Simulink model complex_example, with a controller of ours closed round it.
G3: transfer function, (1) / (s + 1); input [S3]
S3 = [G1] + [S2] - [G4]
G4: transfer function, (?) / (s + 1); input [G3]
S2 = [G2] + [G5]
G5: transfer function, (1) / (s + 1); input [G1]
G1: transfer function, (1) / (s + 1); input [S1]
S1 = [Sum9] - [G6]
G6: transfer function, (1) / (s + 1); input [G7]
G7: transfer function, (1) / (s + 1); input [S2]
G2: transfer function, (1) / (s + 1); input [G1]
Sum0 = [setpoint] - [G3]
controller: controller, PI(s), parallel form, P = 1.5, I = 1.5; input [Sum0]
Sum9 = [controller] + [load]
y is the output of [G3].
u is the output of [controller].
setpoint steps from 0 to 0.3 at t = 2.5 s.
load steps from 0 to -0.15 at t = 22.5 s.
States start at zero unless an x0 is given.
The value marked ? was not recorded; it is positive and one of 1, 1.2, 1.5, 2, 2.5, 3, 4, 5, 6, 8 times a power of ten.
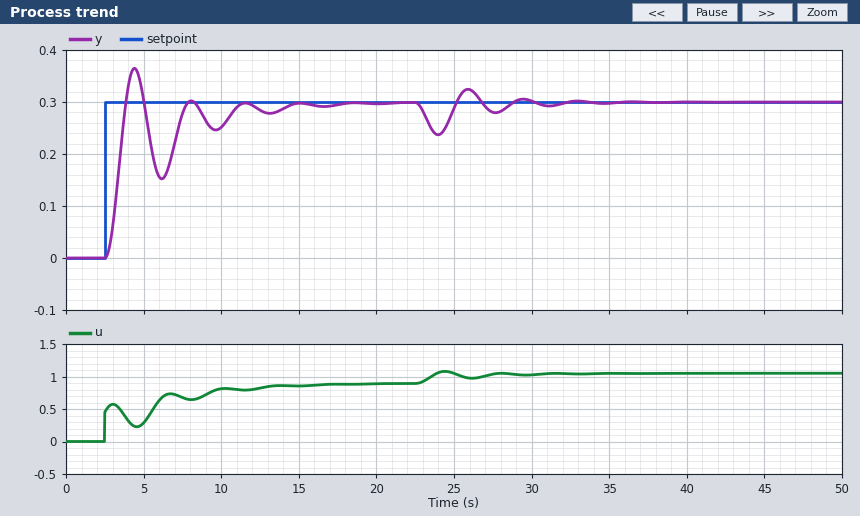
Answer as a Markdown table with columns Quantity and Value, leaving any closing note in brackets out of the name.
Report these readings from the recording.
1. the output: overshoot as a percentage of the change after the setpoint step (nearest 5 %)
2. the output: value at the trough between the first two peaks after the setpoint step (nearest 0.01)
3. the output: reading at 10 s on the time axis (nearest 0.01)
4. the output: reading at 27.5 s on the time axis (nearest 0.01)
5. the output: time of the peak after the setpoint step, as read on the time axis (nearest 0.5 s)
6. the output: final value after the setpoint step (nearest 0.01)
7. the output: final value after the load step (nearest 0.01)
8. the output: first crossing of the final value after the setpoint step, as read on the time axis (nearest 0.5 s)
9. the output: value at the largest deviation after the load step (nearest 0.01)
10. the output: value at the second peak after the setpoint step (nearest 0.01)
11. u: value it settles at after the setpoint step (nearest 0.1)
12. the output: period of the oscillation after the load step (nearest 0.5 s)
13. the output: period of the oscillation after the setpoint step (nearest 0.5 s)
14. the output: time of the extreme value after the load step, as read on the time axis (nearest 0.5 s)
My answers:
| Quantity | Value |
|---|---|
| the output: overshoot as a percentage of the change after the setpoint step | 20 % |
| the output: value at the trough between the first two peaks after the setpoint step | 0.15 |
| the output: reading at 10 s on the time axis | 0.25 |
| the output: reading at 27.5 s on the time axis | 0.28 |
| the output: time of the peak after the setpoint step, as read on the time axis | 4.5 s |
| the output: final value after the setpoint step | 0.30 |
| the output: final value after the load step | 0.30 |
| the output: first crossing of the final value after the setpoint step, as read on the time axis | 4.0 s |
| the output: value at the largest deviation after the load step | 0.24 |
| the output: value at the second peak after the setpoint step | 0.30 |
| u: value it settles at after the setpoint step | 0.9 |
| the output: period of the oscillation after the load step | 3.5 s |
| the output: period of the oscillation after the setpoint step | 3.5 s |
| the output: time of the extreme value after the load step, as read on the time axis | 24.0 s |
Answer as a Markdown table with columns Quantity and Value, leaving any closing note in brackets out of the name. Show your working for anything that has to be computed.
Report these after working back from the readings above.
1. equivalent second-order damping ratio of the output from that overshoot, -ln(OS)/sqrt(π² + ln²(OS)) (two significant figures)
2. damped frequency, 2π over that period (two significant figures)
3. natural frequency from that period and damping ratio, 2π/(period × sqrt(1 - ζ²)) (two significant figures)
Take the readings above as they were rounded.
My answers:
| Quantity | Value |
|---|---|
| equivalent second-order damping ratio of the output from that overshoot, -ln(OS)/sqrt(π² + ln²(OS)) | ln(0.2) = -1.609; 1.609 / sqrt(9.870 + 2.590) = 0.46 |
| damped frequency, 2π over that period | 2π / 3.5 = 1.8 rad/s |
| natural frequency from that period and damping ratio, 2π/(period × sqrt(1 - ζ²)) | 2π / (3.5 × sqrt(1 - 0.46²)) = 2.0 rad/s |
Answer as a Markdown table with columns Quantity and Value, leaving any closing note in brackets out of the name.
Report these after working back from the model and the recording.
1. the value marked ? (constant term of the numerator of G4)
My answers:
| Quantity | Value |
|---|---|
| the value marked ? | 2 |
